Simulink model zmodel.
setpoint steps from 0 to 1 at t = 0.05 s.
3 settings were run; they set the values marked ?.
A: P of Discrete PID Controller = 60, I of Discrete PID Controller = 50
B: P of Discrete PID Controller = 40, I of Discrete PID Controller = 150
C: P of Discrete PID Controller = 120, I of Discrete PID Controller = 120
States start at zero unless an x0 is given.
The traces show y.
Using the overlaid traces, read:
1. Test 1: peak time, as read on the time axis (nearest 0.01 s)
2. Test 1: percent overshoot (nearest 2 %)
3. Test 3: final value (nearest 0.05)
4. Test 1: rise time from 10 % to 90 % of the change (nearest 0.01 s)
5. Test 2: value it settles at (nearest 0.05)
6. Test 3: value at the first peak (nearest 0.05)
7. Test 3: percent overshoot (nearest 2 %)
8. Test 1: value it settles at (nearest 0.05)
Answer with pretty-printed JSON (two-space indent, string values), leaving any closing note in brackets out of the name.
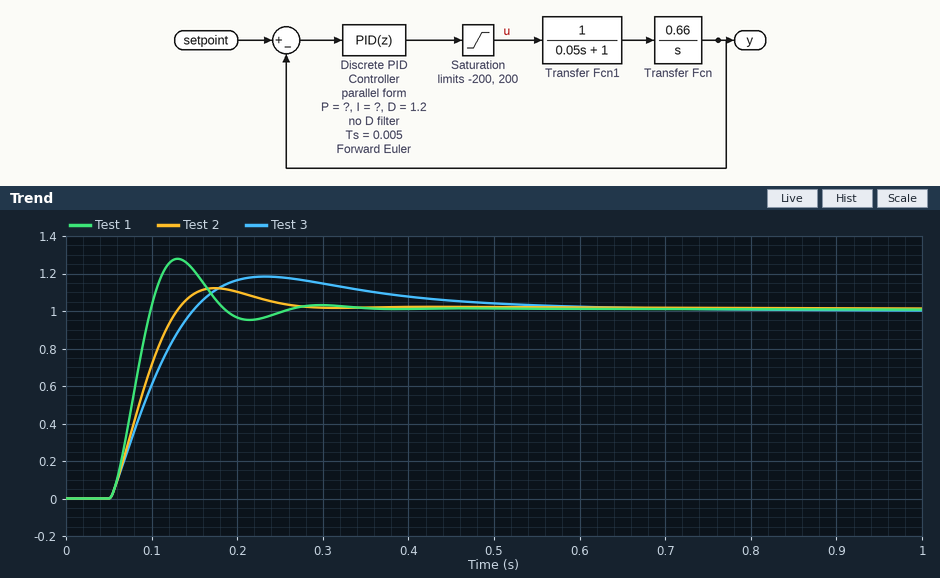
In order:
{
  "Test 1: peak time, as read on the time axis": "0.13 s",
  "Test 1: percent overshoot": "28 %",
  "Test 3: final value": "1.00",
  "Test 1: rise time from 10 % to 90 % of the change": "0.03 s",
  "Test 2: value it settles at": "1.00",
  "Test 3: value at the first peak": "1.20",
  "Test 3: percent overshoot": "18 %",
  "Test 1: value it settles at": "1.00"
}
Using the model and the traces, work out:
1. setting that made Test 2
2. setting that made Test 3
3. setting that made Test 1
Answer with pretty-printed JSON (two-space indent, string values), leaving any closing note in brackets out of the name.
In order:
{
  "setting that made Test 2": "A",
  "setting that made Test 3": "B",
  "setting that made Test 1": "C"
}
